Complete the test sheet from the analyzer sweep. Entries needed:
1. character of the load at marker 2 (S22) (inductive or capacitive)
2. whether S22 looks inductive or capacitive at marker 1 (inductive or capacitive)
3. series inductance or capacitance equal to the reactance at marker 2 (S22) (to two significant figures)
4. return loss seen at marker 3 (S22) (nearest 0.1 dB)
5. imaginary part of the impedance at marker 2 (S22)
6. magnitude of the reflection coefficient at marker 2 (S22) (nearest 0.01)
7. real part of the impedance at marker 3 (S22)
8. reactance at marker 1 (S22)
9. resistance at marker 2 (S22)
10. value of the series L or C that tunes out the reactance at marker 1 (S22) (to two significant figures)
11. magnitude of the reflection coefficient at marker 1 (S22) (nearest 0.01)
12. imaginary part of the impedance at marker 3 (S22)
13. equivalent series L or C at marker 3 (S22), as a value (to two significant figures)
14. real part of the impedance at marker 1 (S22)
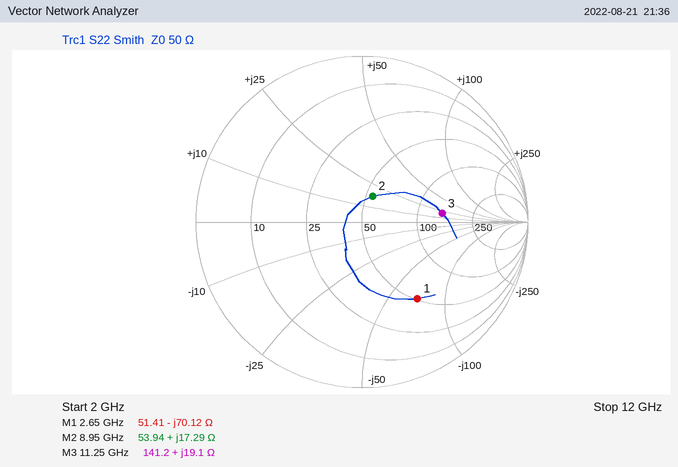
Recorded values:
inductive
capacitive
310 pH
6.3 dB
+17.29 Ω
0.17
141.2 Ω
-70.12 Ω
53.94 Ω
4.2 nH
0.57
+19.1 Ω
270 pH
51.41 Ω
